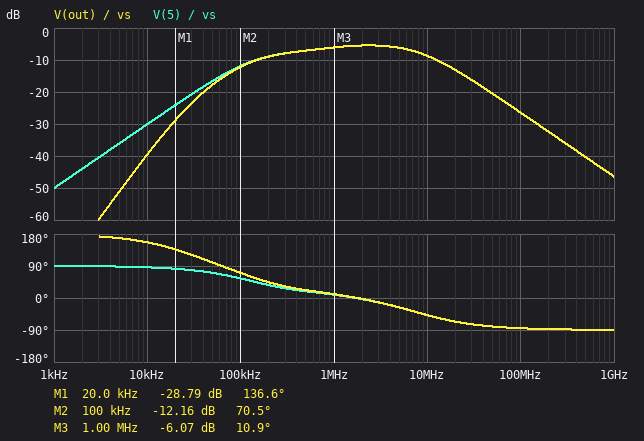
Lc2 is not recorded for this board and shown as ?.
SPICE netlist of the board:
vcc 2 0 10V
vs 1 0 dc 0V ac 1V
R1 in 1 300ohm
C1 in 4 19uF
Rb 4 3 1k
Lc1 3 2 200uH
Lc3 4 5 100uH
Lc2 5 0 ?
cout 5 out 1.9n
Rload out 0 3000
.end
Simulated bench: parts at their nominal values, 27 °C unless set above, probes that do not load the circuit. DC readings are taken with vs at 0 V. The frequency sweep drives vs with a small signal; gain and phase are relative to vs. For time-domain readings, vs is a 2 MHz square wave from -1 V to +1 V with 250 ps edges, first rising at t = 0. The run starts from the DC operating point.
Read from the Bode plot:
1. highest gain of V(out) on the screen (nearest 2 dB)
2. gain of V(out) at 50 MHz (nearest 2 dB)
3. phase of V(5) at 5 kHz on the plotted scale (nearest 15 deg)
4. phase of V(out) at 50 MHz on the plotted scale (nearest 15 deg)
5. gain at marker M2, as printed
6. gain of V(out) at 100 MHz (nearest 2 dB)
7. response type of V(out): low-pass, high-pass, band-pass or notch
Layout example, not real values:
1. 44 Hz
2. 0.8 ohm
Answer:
1. -6 dB
2. -20 dB
3. 90 deg
4. -75 deg
5. -12.16 dB
6. -26 dB
7. band-pass
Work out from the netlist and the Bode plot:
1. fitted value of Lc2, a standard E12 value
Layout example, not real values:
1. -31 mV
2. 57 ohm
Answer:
1. 150 µH
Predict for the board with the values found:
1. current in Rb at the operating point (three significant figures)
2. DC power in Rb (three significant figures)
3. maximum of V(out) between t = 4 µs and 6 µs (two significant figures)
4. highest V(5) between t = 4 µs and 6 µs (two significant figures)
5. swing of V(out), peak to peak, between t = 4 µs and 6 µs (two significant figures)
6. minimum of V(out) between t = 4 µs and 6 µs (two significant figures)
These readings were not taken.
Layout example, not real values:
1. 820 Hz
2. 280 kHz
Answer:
1. 10.0 mA
2. 100 mW
3. 580 mV
4. 620 mV
5. 1.2 V
6. -650 mV
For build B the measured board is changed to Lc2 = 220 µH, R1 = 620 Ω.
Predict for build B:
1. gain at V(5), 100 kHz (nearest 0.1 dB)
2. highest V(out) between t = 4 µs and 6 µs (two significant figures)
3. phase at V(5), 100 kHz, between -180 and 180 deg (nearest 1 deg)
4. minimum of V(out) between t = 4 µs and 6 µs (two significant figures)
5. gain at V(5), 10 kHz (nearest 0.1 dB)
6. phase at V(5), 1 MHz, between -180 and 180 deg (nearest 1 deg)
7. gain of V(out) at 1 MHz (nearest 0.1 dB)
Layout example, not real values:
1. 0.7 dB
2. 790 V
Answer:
1. -14.3 dB
2. 640 mV
3. 61 deg
4. -700 mV
5. -33.0 dB
6. 17 deg
7. -6.7 dB
